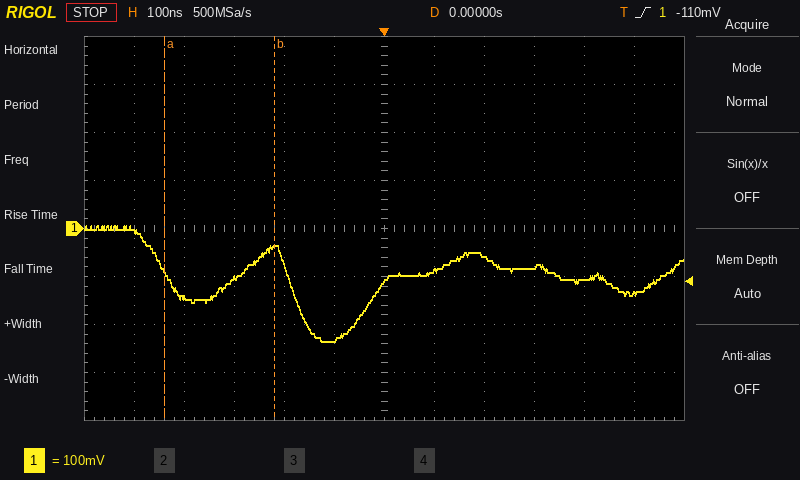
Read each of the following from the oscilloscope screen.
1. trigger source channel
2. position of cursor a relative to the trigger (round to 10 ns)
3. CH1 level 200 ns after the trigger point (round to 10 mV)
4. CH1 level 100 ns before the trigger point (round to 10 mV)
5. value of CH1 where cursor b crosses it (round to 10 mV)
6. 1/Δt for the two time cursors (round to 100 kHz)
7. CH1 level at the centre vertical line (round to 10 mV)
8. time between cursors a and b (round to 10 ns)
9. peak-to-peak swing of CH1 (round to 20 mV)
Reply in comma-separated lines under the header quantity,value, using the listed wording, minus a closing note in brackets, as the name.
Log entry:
quantity,value
trigger source channel,CH1
position of cursor a relative to the trigger,-440 ns
CH1 level 200 ns after the trigger point,-60 mV
CH1 level 100 ns before the trigger point,-230 mV
value of CH1 where cursor b crosses it,-40 mV
1/Δt for the two time cursors,4.5 MHz
CH1 level at the centre vertical line,-110 mV
time between cursors a and b,220 ns
peak-to-peak swing of CH1,240 mV
